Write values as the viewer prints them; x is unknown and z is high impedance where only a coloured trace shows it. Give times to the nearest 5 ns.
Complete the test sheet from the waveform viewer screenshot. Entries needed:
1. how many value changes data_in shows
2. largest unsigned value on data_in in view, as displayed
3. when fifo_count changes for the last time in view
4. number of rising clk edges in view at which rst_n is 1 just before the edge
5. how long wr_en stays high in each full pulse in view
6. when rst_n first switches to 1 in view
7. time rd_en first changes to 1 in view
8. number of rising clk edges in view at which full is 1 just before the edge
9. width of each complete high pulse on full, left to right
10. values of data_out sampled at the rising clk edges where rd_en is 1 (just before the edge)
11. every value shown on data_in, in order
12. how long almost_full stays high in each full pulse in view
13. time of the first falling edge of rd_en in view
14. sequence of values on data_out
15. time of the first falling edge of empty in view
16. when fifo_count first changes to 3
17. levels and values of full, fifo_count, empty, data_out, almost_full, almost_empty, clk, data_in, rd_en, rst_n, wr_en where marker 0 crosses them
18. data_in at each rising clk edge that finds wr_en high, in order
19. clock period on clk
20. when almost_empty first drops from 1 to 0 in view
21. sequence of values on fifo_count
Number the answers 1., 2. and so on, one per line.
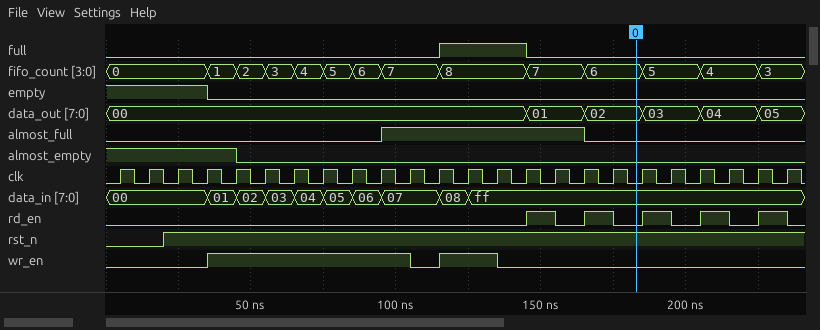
1. 9
2. ff
3. 225 ns
4. 22
5. 70 ns, 20 ns
6. 20 ns
7. 145 ns
8. 3
9. 30 ns
10. 01, 02, 03, 04, 05
11. 00, 01, 02, 03, 04, 05, 06, 07, 08, ff
12. 70 ns
13. 155 ns
14. 00, 01, 02, 03, 04, 05
15. 35 ns
16. 55 ns
17. full=0, fifo_count=6, empty=0, data_out=02, almost_full=0, almost_empty=0, clk=0, data_in=ff, rd_en=0, rst_n=1, wr_en=0
18. 01, 02, 03, 04, 05, 06, 07, 08, ff
19. 10 ns
20. 45 ns
21. 0, 1, 2, 3, 4, 5, 6, 7, 8, 7, 6, 5, 4, 3
